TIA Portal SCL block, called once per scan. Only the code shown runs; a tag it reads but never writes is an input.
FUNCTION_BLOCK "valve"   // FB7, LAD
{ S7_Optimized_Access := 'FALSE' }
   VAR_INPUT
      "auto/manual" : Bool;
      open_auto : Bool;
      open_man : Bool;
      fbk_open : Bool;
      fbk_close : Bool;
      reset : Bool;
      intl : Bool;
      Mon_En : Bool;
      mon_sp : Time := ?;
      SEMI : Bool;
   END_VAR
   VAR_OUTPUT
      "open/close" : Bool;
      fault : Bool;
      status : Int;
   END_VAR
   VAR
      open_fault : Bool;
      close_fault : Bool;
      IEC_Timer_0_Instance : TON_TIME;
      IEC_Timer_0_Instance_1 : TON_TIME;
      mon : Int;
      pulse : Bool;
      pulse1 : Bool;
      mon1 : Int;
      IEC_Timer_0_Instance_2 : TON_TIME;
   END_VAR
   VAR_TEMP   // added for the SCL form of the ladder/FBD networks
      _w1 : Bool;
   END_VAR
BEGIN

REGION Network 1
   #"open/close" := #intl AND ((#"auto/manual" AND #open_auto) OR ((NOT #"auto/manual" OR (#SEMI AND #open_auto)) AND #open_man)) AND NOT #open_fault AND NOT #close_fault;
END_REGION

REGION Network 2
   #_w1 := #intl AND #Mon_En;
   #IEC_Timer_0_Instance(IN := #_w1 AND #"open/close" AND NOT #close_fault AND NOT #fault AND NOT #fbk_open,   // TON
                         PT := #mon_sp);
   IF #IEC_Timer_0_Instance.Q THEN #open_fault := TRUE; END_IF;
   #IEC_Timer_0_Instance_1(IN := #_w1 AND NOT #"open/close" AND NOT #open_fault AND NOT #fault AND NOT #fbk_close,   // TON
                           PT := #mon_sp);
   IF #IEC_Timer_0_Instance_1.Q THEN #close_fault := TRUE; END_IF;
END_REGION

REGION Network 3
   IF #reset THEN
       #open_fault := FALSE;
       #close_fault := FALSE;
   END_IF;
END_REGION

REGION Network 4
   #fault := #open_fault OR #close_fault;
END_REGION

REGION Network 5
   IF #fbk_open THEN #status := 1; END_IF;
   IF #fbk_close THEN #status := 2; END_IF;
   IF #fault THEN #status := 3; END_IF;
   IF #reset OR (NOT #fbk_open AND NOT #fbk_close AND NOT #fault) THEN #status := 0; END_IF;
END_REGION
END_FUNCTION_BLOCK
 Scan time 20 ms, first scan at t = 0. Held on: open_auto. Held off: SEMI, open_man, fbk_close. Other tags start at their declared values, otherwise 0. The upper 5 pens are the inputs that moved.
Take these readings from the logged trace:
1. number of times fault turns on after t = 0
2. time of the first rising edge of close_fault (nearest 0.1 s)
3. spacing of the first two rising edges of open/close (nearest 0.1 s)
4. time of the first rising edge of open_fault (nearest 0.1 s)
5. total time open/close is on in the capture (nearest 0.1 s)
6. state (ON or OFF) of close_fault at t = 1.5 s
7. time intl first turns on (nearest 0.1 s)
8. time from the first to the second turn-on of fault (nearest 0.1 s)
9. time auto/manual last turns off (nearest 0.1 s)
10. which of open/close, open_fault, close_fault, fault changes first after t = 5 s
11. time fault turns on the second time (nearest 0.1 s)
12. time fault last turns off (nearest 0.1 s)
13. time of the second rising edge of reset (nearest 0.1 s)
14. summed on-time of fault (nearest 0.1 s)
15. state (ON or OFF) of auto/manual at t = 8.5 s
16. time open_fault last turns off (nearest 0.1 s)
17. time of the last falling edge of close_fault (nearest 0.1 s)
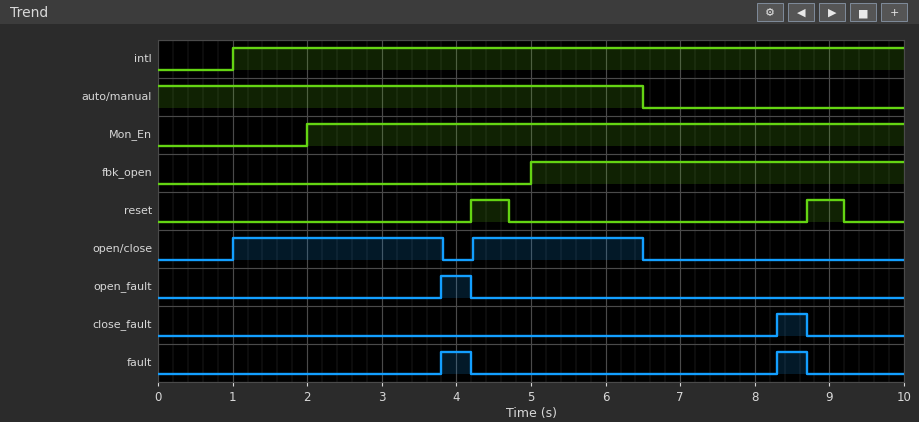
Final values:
2
8.3 s
3.2 s
3.8 s
5.1 s
OFF
1.0 s
4.5 s
6.5 s
open/close
8.3 s
8.7 s
8.7 s
0.8 s
OFF
4.2 s
8.7 s
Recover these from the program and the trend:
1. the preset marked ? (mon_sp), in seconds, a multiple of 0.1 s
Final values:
1.8 s
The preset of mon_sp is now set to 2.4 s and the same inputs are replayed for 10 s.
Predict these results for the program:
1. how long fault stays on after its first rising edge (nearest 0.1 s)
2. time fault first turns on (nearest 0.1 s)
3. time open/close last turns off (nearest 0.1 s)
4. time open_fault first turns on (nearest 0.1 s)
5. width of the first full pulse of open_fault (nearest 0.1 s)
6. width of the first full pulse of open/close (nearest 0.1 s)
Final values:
4.0 s
4.7 s
4.7 s
4.7 s
4.0 s
3.7 s
